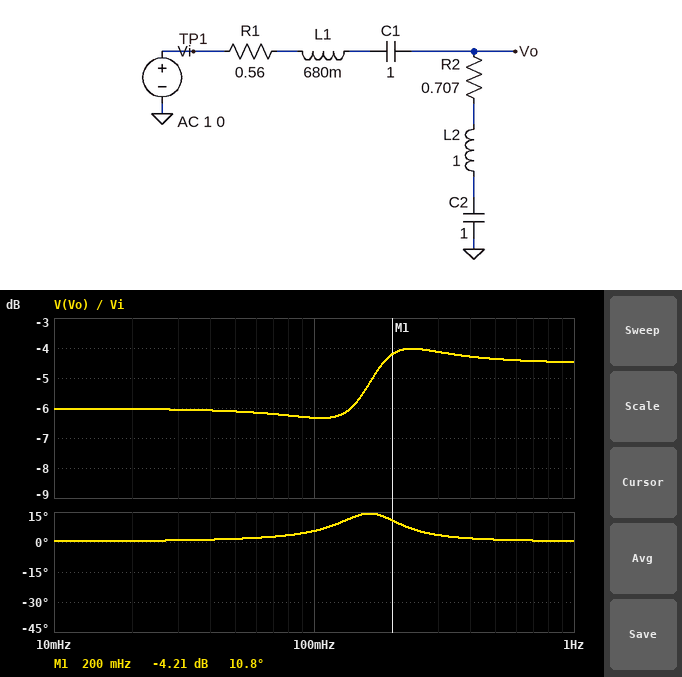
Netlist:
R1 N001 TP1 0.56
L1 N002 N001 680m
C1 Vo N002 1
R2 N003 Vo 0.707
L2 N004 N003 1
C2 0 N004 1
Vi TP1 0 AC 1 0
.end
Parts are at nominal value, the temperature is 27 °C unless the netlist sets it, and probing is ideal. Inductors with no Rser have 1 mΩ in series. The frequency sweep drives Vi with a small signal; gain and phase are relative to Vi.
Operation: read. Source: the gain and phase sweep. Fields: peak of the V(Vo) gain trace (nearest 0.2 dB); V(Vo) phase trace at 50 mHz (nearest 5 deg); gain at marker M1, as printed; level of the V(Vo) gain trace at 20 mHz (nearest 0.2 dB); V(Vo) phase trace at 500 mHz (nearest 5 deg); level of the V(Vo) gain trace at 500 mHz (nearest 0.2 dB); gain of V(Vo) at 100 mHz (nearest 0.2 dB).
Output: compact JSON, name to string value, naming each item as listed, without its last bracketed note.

{"peak of the V(Vo) gain trace": "-4.0 dB", "V(Vo) phase trace at 50 mHz": "0 deg", "gain at marker M1, as printed": "-4.21 dB", "level of the V(Vo) gain trace at 20 mHz": "-6.0 dB", "V(Vo) phase trace at 500 mHz": "0 deg", "level of the V(Vo) gain trace at 500 mHz": "-4.4 dB", "gain of V(Vo) at 100 mHz": "-6.4 dB"}
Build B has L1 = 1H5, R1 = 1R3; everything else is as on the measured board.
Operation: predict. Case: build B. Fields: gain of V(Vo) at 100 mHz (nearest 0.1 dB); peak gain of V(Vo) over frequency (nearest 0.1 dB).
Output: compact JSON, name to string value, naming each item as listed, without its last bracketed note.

{"gain of V(Vo) at 100 mHz": "-6.7 dB", "peak gain of V(Vo) over frequency": "-6.0 dB"}
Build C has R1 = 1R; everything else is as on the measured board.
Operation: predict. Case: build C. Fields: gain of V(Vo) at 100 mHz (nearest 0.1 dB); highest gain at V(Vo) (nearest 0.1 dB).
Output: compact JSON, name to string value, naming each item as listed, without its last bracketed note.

{"gain of V(Vo) at 100 mHz": "-7.2 dB", "highest gain at V(Vo)": "-4.5 dB"}
